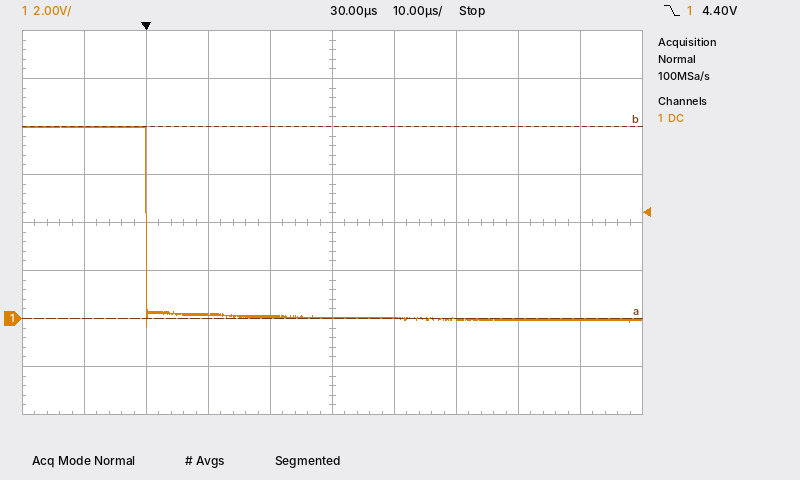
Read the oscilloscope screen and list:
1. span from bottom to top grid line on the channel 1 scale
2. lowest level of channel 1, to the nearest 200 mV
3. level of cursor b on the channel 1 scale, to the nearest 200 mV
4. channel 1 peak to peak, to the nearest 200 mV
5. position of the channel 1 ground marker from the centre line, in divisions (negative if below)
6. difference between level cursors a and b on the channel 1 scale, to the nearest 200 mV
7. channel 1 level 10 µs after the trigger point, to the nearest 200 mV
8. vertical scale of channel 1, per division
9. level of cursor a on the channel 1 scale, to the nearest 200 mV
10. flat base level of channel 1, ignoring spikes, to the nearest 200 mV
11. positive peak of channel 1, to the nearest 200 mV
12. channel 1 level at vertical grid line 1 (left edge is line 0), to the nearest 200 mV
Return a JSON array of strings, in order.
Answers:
["16 V", "-400 mV", "8.0 V", "8.4 V", "-2.0 div", "8.0 V", "200 mV", "2 V", "0.0 V", "0.0 V", "8.0 V", "8.0 V"]
